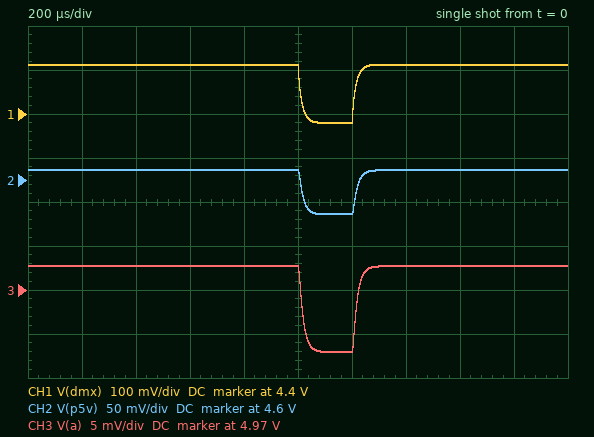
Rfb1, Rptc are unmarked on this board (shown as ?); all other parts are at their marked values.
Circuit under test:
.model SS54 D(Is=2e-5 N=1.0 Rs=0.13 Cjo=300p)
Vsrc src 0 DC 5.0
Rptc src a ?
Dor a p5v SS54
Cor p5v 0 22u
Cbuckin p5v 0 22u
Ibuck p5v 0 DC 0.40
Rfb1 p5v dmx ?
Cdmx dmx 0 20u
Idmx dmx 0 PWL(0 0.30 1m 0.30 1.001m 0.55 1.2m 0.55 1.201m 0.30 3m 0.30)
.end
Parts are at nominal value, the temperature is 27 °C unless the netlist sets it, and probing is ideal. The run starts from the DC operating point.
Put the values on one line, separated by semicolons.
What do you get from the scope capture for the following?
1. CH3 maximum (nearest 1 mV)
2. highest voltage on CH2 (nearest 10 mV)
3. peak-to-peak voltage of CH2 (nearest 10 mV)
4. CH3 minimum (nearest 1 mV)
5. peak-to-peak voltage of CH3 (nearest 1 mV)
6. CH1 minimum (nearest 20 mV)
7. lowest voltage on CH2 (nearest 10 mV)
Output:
4.973 V; 4.61 V; 50 mV; 4.963 V; 10 mV; 4.38 V; 4.56 V
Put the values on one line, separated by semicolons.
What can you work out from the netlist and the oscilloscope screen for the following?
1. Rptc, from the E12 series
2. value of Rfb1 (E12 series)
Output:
0.039 Ω; 0.33 Ω
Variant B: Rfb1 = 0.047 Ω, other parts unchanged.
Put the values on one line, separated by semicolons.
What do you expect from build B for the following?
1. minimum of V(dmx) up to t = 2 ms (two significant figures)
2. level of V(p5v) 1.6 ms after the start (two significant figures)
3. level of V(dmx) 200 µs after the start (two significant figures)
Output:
4.5 V; 4.6 V; 4.6 V
